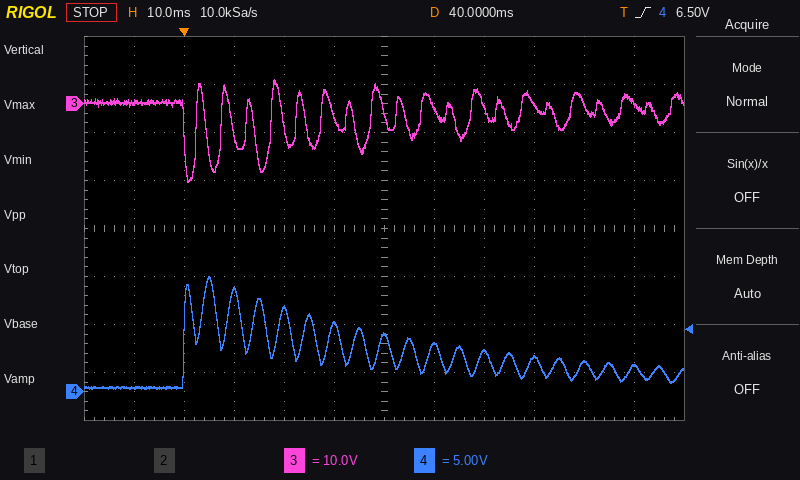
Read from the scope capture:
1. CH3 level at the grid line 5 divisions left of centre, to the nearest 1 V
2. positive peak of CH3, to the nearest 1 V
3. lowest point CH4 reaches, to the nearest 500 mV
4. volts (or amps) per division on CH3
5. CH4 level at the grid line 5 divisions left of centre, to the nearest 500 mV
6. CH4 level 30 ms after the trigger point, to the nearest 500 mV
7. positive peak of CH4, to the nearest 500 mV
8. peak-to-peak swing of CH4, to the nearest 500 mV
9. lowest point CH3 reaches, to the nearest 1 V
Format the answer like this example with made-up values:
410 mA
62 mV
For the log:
0 V
5 V
500 mV
10 V
500 mV
7.0 V
12.0 V
11.5 V
-16 V
